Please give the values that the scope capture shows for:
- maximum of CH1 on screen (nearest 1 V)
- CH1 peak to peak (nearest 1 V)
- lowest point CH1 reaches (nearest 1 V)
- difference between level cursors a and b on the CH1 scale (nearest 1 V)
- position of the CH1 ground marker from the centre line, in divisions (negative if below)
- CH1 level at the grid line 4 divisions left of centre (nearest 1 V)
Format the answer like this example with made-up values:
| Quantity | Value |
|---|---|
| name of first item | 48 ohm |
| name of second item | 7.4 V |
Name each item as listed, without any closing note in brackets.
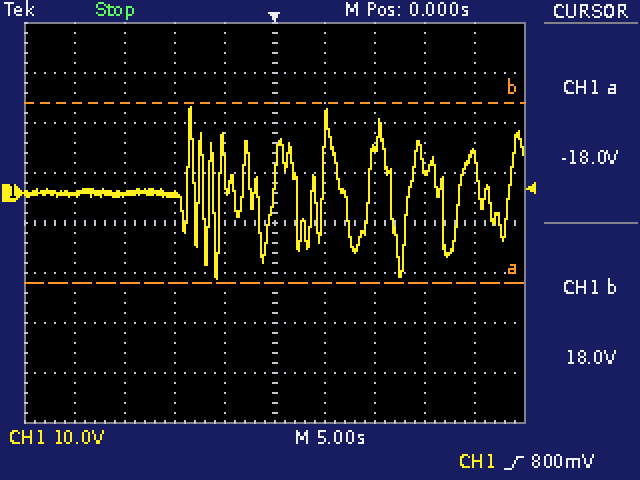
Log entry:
| Quantity | Value |
|---|---|
| maximum of CH1 on screen | 17 V |
| CH1 peak to peak | 34 V |
| lowest point CH1 reaches | -17 V |
| difference between level cursors a and b on the CH1 scale | 36 V |
| position of the CH1 ground marker from the centre line, in divisions | +0.6 div |
| CH1 level at the grid line 4 divisions left of centre | 0 V |
